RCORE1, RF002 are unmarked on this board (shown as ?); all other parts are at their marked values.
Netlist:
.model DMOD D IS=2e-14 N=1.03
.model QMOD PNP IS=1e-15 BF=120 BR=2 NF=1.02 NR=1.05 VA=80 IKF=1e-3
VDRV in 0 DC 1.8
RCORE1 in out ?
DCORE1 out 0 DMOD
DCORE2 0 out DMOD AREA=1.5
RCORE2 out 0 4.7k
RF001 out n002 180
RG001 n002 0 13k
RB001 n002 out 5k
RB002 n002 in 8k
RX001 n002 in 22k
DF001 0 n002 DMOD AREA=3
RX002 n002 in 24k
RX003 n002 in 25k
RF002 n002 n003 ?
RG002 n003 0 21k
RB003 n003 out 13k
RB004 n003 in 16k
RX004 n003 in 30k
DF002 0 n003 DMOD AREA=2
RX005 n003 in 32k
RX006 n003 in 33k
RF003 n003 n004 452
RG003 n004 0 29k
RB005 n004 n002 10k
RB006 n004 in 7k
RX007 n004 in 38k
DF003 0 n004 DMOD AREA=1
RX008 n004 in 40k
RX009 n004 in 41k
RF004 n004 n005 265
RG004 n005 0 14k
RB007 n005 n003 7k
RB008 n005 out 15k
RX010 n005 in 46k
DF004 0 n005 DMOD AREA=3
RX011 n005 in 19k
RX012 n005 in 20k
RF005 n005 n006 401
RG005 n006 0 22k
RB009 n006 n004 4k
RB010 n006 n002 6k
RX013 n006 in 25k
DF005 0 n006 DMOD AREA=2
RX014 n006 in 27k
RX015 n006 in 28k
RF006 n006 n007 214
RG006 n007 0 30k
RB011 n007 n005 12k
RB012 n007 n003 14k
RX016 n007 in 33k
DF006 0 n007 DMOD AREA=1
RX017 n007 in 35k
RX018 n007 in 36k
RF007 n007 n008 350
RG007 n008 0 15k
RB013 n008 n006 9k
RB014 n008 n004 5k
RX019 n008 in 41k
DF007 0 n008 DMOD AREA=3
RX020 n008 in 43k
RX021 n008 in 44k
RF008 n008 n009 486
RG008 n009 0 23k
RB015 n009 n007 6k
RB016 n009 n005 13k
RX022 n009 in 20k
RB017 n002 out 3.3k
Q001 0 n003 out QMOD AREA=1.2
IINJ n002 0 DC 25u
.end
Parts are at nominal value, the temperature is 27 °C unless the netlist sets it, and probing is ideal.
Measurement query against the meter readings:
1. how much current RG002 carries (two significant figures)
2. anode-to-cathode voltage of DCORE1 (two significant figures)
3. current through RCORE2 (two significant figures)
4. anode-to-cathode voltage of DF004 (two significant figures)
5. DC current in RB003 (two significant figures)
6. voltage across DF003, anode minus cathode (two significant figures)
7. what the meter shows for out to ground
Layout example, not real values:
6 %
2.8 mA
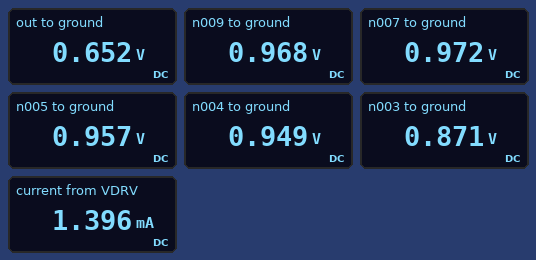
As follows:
41 µA
650 mV
140 µA
-960 mV
17 µA
-950 mV
0.652 V
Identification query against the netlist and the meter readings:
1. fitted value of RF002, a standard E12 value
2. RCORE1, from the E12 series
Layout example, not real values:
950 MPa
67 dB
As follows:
470 Ω
2.7 kΩ
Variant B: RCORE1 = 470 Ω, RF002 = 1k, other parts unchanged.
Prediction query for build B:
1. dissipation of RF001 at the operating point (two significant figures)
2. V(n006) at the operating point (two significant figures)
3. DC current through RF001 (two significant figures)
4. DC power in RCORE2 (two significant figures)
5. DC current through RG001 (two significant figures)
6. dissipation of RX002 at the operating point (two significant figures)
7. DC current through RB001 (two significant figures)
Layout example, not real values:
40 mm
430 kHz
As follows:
30 µW
1.0 V
410 µA
99 µW
58 µA
45 µW
15 µA
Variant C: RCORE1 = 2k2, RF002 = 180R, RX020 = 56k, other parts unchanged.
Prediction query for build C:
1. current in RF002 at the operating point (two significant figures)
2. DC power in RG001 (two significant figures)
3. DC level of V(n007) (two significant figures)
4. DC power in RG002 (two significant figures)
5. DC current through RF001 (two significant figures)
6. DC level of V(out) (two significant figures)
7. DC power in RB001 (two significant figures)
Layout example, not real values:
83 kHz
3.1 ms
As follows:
340 µA
43 µW
940 mV
31 µW
520 µA
660 mV
1.8 µW
